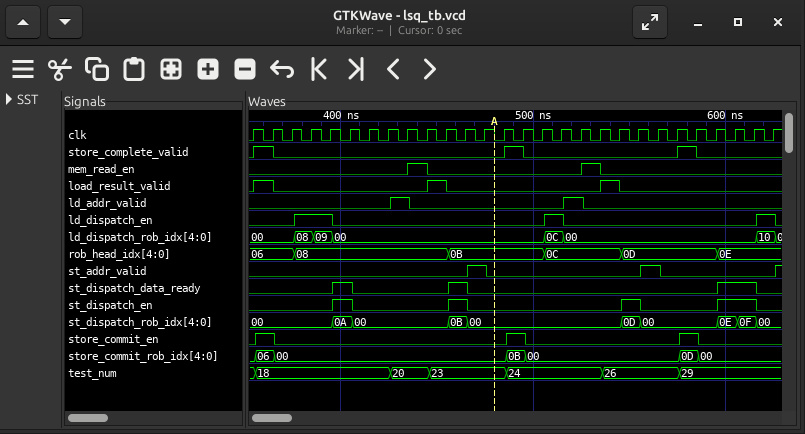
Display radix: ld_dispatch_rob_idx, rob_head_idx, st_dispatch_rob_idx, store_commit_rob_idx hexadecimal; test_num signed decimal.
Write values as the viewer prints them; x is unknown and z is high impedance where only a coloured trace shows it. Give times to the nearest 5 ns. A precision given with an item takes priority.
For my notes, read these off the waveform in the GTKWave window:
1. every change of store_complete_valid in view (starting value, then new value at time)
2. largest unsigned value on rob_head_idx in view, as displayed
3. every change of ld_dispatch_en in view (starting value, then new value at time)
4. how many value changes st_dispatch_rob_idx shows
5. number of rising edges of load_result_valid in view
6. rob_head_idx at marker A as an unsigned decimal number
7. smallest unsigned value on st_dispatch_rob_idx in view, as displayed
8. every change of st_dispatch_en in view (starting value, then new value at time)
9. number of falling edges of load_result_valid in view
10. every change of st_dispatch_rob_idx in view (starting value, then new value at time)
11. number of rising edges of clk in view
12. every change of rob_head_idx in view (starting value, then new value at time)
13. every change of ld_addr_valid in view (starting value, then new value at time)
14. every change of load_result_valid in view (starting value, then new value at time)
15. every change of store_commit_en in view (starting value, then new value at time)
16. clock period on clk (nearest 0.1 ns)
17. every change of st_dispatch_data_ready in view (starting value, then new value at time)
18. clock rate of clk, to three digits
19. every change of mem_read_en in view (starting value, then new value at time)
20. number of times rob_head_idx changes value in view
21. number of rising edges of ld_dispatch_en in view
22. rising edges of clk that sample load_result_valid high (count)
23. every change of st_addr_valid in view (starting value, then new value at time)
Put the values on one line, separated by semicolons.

0, 1 at 355 ns, 0 at 365 ns, 1 at 485 ns, 0 at 495 ns, 1 at 575 ns, 0 at 585 ns; 0E; 0, 1 at 375 ns, 0 at 395 ns, 1 at 505 ns, 0 at 515 ns, 1 at 615 ns, 0 at 625 ns; 9; 3; 11; 00; 0, 1 at 395 ns, 0 at 405 ns, 1 at 455 ns, 0 at 465 ns, 1 at 545 ns, 0 at 555 ns, 1 at 595 ns, 0 at 615 ns; 3; 00, 0A at 395 ns, 00 at 405 ns, 0B at 455 ns, 00 at 465 ns, 0D at 545 ns, 00 at 555 ns, 0E at 595 ns, 0F at 605 ns, 00 at 615 ns; 28; 06, 08 at 375 ns, 0B at 455 ns, 0C at 505 ns, 0D at 545 ns, 0E at 595 ns; 0, 1 at 425 ns, 0 at 435 ns, 1 at 515 ns, 0 at 525 ns; 0, 1 at 355 ns, 0 at 365 ns, 1 at 445 ns, 0 at 455 ns, 1 at 535 ns, 0 at 545 ns; 0, 1 at 355 ns, 0 at 365 ns, 1 at 485 ns, 0 at 495 ns, 1 at 575 ns, 0 at 585 ns; 10 ns; 0, 1 at 395 ns, 0 at 405 ns, 1 at 455 ns, 0 at 465 ns, 1 at 595 ns, 0 at 615 ns; 100 MHz; 0, 1 at 435 ns, 0 at 445 ns, 1 at 525 ns, 0 at 535 ns; 5; 3; 3; 0, 1 at 465 ns, 0 at 475 ns, 1 at 555 ns, 0 at 565 ns, 1 at 625 ns
